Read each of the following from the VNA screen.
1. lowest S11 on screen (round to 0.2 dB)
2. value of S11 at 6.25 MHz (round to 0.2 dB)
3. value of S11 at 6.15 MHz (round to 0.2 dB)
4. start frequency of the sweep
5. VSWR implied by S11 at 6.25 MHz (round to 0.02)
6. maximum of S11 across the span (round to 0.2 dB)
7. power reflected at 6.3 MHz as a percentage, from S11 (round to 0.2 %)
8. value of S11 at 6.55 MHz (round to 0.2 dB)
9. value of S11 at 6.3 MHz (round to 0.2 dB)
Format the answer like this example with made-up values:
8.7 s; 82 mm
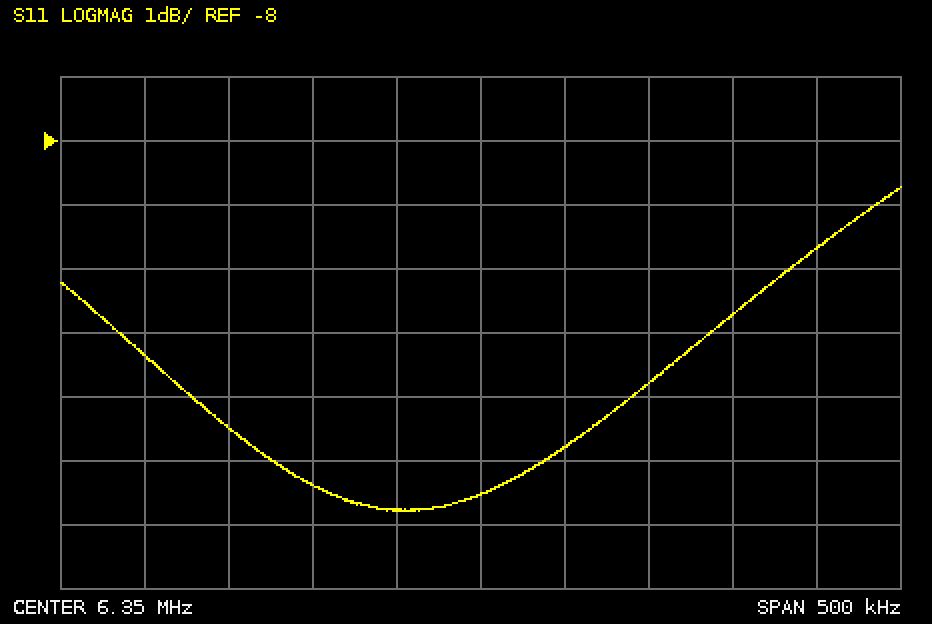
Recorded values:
-13.8 dB; -13.4 dB; -11.4 dB; 6.1 MHz; 1.54; -8.8 dB; 4.2 %; -9.6 dB; -13.8 dB
